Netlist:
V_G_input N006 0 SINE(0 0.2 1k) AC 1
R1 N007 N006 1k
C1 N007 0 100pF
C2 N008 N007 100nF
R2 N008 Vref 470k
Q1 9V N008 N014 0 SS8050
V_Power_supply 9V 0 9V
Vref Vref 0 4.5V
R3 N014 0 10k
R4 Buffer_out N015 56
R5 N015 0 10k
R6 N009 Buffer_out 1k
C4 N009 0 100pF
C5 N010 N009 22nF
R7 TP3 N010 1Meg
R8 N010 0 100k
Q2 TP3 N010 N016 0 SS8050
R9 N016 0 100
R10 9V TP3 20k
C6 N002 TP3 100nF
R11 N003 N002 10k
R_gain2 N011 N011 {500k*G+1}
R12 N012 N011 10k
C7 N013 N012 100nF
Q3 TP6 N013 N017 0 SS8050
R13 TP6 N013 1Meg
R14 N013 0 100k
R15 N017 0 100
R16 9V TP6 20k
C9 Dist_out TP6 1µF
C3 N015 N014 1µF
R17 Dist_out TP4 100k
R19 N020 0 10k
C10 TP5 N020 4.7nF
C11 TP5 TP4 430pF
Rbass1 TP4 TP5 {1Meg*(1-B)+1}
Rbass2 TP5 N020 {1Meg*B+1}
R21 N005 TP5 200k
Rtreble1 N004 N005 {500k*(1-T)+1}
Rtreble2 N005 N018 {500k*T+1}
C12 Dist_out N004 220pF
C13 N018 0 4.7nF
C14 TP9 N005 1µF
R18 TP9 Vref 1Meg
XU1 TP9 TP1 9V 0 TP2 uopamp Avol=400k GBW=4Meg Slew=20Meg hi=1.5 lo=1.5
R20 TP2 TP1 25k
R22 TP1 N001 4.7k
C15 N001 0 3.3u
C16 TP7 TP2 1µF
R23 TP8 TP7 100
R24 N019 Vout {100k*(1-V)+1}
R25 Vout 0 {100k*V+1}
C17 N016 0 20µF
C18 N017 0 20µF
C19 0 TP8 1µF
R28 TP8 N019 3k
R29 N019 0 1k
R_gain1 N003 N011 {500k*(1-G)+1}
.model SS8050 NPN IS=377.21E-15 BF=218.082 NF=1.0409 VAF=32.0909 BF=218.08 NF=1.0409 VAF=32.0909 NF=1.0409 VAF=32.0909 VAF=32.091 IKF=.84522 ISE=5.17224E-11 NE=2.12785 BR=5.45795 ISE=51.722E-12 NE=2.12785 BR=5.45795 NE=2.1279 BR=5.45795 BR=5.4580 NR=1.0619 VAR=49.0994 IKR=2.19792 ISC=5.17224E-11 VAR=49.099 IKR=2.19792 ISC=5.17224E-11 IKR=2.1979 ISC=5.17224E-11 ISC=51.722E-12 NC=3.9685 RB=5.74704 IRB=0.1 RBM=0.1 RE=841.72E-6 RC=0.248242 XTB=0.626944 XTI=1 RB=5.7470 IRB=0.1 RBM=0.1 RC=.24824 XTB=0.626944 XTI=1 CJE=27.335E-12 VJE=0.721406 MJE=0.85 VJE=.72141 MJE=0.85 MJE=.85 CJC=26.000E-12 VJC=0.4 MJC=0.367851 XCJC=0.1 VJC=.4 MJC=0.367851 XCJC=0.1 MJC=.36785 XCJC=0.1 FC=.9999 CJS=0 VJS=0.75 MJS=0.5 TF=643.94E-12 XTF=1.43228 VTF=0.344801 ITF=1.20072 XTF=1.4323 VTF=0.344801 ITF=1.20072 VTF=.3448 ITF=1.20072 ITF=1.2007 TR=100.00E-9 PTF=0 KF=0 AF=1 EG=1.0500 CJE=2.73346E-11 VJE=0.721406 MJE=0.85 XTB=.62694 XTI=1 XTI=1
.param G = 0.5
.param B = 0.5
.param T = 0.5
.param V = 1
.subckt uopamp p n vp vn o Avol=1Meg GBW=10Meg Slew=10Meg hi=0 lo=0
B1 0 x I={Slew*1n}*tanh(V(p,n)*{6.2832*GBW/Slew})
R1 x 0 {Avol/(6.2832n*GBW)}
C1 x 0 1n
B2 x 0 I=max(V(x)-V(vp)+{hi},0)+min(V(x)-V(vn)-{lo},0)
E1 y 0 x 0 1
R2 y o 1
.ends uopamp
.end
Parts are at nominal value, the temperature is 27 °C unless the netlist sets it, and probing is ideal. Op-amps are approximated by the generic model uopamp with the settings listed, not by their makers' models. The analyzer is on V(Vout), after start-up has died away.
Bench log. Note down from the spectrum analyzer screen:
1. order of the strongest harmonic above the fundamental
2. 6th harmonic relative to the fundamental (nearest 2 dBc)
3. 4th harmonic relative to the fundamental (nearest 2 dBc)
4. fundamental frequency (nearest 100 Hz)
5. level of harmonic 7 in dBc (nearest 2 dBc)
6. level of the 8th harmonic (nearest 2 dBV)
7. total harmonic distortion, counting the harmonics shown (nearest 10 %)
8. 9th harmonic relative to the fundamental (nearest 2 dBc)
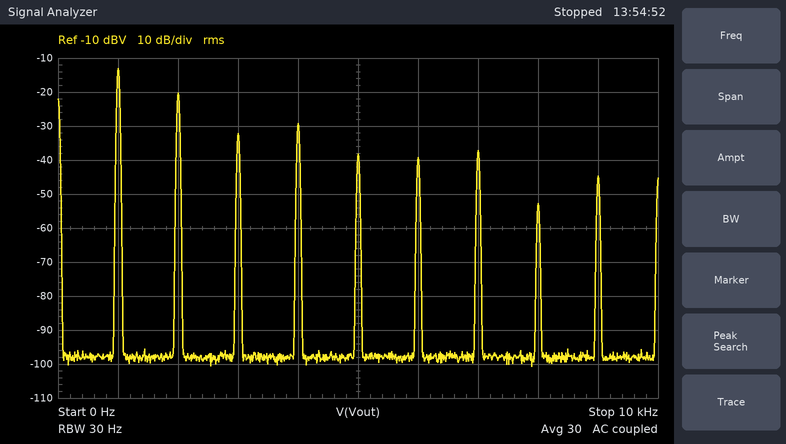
2
-26 dBc
-16 dBc
1.0 kHz
-24 dBc
-52 dBV
50 %
-32 dBc
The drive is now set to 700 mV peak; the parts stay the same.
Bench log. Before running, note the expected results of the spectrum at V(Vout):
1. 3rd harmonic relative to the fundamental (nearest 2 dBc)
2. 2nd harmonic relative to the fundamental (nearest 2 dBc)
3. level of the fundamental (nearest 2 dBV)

-14 dBc
-10 dBc
-12 dBV
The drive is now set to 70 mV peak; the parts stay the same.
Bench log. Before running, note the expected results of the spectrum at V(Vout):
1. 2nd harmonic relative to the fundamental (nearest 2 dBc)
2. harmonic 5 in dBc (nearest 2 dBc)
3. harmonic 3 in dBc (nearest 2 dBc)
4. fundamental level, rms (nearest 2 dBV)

-24 dBc
-30 dBc
-14 dBc
-12 dBV
